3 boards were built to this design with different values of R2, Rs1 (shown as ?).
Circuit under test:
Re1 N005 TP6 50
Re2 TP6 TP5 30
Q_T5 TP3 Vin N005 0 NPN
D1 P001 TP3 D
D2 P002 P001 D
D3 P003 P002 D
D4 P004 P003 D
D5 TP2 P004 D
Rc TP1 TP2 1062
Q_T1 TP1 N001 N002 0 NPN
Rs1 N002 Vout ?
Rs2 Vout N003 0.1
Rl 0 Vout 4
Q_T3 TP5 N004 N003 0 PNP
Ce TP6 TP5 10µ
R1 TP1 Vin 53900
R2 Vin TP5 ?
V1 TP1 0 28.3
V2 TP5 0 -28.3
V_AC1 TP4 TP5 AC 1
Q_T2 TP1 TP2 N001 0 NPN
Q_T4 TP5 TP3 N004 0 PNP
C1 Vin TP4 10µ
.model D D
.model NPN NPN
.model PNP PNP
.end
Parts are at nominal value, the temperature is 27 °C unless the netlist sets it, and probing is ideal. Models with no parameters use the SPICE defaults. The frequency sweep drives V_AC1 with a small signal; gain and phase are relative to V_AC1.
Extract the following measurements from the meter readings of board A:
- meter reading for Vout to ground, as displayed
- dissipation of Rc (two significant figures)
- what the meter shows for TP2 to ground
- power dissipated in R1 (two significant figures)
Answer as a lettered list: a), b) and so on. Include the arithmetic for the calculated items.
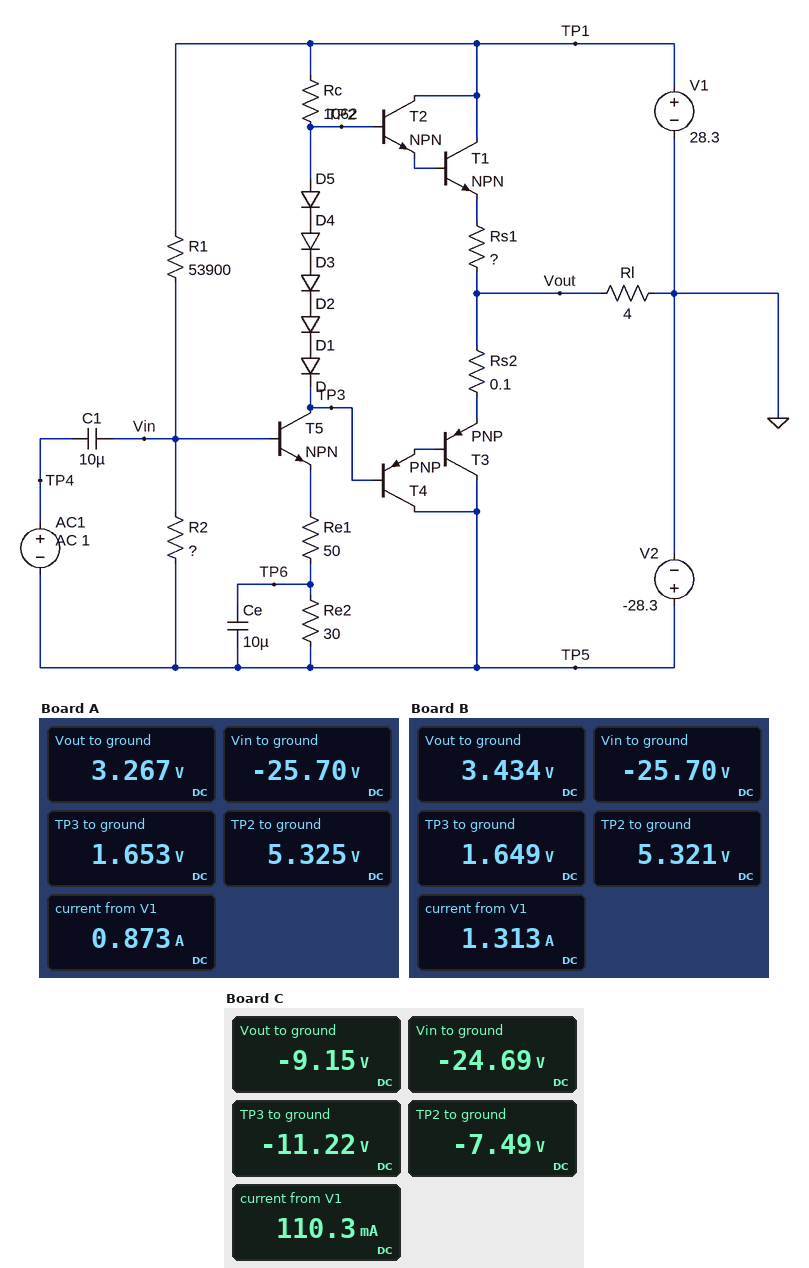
a) 3.267 V
b) (28.3 V - 5.325 V)^2 / 1.062 kΩ = 500 mW
c) 5.325 V
d) (28.3 V - (-25.7 V))^2 / 53.9 kΩ = 54 mW
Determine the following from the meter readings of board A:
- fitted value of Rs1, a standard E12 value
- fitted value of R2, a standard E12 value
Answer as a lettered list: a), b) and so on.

a) 0.33 Ω
b) 3.3 kΩ
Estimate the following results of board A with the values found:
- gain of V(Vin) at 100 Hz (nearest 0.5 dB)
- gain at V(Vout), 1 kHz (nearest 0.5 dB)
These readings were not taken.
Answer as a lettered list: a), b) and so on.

a) 0 dB
b) 24.0 dB
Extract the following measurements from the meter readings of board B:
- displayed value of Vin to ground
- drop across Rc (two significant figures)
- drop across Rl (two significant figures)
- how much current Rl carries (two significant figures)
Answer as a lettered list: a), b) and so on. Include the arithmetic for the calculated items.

a) -25.70 V
b) 28.3 V - 5.321 V = 23 V
c) 3.434 V = 3.4 V
d) (3.434 V) / 4 Ω = 860 mA
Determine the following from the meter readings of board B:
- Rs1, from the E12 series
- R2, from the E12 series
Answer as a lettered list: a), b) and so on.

a) 0.068 Ω
b) 3.3 kΩ
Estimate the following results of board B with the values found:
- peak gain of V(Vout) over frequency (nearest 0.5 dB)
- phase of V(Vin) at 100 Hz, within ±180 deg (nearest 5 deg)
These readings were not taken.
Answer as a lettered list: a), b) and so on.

a) 26.0 dB
b) 5 deg
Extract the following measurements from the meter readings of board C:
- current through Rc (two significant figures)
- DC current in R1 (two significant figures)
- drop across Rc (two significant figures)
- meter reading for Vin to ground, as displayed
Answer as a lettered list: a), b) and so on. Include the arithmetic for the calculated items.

a) (28.3 V - (-7.49 V)) / 1.062 kΩ = 34 mA
b) (28.3 V - (-24.69 V)) / 53.9 kΩ = 980 µA
c) 28.3 V - (-7.49 V) = 36 V
d) -24.69 V
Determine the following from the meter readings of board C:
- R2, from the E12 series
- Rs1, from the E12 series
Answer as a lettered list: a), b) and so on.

a) 5.6 kΩ
b) 0.15 Ω
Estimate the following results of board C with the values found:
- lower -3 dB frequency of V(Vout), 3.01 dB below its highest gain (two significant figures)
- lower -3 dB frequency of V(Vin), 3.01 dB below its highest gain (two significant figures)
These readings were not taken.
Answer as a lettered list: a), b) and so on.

a) 390 Hz
b) 5.1 Hz
